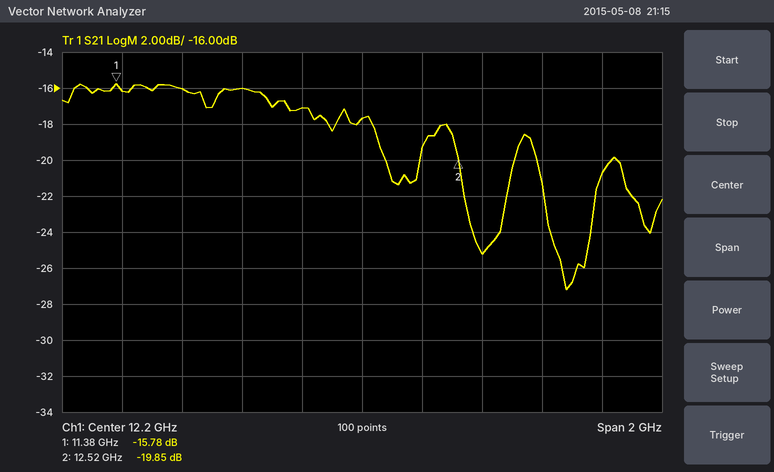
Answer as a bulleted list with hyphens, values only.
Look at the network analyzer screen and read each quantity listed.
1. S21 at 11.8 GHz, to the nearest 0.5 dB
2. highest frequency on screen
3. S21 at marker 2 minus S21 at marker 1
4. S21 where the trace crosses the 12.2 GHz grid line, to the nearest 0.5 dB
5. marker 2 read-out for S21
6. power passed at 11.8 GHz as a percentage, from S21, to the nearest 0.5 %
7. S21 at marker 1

- -16.0 dB
- 13.2 GHz
- -4.07 dB
- -17.5 dB
- -19.85 dB
- 2.5 %
- -15.78 dB
